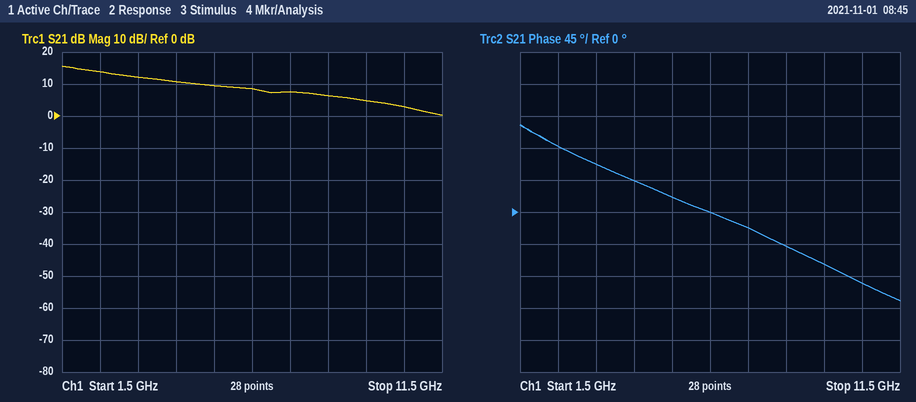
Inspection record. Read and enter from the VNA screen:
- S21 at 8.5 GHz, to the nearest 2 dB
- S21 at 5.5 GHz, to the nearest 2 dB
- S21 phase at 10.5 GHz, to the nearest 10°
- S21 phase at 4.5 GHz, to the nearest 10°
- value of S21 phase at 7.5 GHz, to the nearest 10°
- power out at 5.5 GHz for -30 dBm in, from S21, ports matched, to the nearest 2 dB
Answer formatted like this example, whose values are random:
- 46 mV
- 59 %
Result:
- 6 dB
- 10 dB
- -100°
- 40°
- -20°
- -20 dBm
